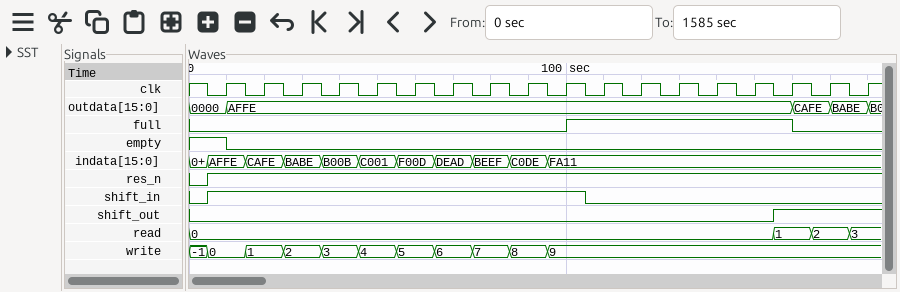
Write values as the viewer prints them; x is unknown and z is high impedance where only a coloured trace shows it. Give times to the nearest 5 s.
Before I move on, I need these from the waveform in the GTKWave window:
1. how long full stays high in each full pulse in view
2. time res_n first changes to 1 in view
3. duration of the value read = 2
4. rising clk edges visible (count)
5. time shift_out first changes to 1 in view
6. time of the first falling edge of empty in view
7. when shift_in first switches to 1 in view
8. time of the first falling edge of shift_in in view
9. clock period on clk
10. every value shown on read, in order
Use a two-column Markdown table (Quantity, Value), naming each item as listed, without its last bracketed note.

| Quantity | Value |
|---|---|
| how long full stays high in each full pulse in view | 60 s |
| time res_n first changes to 1 in view | 5 s |
| duration of the value read = 2 | 10 s |
| rising clk edges visible | 18 |
| time shift_out first changes to 1 in view | 155 s |
| time of the first falling edge of empty in view | 10 s |
| when shift_in first switches to 1 in view | 5 s |
| time of the first falling edge of shift_in in view | 105 s |
| clock period on clk | 10 s |
| every value shown on read, in order | 0, 1, 2, 3 |
